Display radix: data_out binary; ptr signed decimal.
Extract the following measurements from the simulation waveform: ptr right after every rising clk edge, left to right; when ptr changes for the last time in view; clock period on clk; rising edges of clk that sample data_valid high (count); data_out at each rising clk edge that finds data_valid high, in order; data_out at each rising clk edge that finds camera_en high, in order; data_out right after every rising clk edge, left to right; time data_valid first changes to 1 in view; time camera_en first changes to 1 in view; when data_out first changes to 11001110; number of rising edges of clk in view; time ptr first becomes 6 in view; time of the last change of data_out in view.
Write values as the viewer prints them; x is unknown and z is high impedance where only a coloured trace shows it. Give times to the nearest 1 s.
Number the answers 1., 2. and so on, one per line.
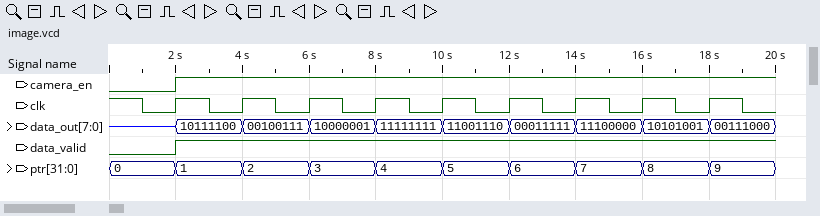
1. 1, 2, 3, 4, 5, 6, 7, 8, 9
2. 18 s
3. 2 s
4. 8
5. 10111100, 00100111, 10000001, 11111111, 11001110, 00011111, 11100000, 10101001
6. 10111100, 00100111, 10000001, 11111111, 11001110, 00011111, 11100000, 10101001
7. 10111100, 00100111, 10000001, 11111111, 11001110, 00011111, 11100000, 10101001, 00111000
8. 2 s
9. 2 s
10. 10 s
11. 9
12. 12 s
13. 18 s
